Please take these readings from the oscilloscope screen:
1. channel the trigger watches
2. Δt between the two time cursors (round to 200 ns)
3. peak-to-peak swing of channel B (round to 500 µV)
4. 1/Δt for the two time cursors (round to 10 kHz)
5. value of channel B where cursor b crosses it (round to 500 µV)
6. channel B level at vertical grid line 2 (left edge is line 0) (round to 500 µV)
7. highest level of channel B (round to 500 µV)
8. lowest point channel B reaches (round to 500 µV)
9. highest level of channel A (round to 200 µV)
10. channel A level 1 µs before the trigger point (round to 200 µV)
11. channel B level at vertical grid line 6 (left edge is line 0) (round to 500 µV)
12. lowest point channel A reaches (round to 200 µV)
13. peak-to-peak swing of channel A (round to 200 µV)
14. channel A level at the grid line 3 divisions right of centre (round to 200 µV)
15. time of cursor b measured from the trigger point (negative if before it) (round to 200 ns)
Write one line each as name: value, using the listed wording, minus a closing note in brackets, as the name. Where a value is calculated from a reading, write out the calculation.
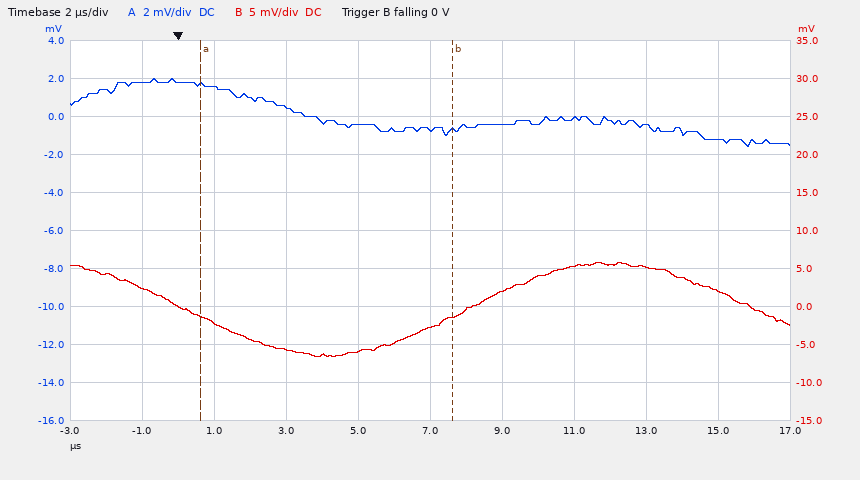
channel the trigger watches: channel B
Δt between the two time cursors: 7.0 µs
peak-to-peak swing of channel B: 6.0 mV − (-6.5 mV) = 12.5 mV
1/Δt for the two time cursors: 1 / 7.0 µs ≈ 140 kHz
value of channel B where cursor b crosses it: -1.5 mV
channel B level at vertical grid line 2 (left edge is line 0): -2.0 mV
highest level of channel B: 6.0 mV
lowest point channel B reaches: -6.5 mV
highest level of channel A: 2.0 mV
channel A level 1 µs before the trigger point: 1.8 mV
channel B level at vertical grid line 6 (left edge is line 0): 2.0 mV
lowest point channel A reaches: -1.6 mV
peak-to-peak swing of channel A: 2.0 mV − (-1.6 mV) = 3.6 mV
channel A level at the grid line 3 divisions right of centre: -400 µV
time of cursor b measured from the trigger point (negative if before it): +7.6 µs
